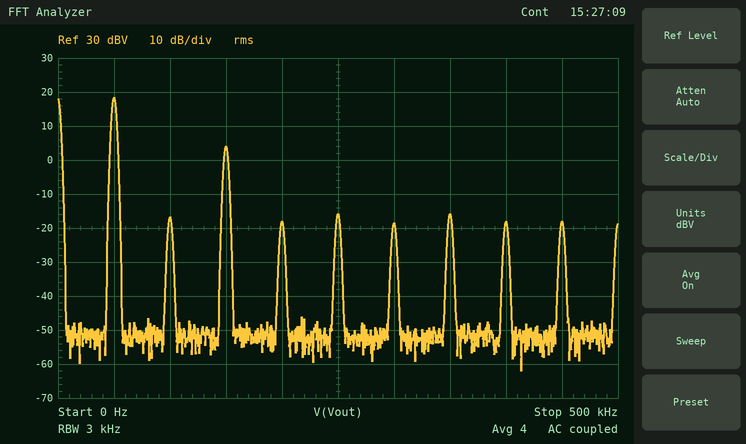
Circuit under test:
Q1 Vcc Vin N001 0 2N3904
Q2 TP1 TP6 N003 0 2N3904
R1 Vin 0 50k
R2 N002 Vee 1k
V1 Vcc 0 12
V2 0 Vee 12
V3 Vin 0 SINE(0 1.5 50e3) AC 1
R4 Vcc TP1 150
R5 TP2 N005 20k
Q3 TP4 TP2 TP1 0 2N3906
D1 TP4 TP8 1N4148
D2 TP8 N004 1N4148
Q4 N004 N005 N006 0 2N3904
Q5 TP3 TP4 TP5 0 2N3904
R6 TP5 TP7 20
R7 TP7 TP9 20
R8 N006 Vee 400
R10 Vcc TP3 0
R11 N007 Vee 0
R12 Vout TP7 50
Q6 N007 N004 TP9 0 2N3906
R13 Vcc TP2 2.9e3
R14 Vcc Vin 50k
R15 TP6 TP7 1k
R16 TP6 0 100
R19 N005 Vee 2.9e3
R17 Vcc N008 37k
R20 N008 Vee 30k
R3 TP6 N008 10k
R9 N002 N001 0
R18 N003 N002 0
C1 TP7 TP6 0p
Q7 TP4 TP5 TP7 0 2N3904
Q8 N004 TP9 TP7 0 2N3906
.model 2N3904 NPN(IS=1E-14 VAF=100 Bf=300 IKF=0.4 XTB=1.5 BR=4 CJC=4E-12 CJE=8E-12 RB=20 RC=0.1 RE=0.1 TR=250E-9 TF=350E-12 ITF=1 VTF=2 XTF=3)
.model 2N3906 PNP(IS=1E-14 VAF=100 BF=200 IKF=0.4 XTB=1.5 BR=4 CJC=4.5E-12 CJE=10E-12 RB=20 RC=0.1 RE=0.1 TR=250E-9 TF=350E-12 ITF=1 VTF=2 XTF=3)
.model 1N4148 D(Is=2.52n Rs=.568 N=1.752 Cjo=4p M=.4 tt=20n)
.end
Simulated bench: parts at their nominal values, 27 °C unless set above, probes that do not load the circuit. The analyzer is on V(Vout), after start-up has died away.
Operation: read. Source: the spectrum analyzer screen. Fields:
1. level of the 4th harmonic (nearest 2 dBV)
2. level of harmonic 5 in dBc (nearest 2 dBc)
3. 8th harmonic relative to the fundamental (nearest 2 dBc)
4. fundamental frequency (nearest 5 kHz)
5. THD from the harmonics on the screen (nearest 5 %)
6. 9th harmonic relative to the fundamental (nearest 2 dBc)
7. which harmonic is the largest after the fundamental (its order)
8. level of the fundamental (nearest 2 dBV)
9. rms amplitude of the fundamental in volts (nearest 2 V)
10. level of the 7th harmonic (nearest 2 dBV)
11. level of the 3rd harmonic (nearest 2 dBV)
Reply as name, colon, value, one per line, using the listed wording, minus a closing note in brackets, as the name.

level of the 4th harmonic: -18 dBV
level of harmonic 5 in dBc: -34 dBc
8th harmonic relative to the fundamental: -36 dBc
fundamental frequency: 50 kHz
THD from the harmonics on the screen: 20 %
9th harmonic relative to the fundamental: -36 dBc
which harmonic is the largest after the fundamental: 3
level of the fundamental: 18 dBV
rms amplitude of the fundamental in volts: 8 V
level of the 7th harmonic: -16 dBV
level of the 3rd harmonic: 4 dBV
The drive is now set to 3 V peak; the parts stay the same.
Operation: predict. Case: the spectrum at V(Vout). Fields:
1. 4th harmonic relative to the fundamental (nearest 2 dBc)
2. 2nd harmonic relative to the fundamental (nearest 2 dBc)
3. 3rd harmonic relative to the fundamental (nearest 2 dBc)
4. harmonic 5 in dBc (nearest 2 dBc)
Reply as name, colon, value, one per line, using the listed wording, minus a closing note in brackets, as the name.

4th harmonic relative to the fundamental: -26 dBc
2nd harmonic relative to the fundamental: -26 dBc
3rd harmonic relative to the fundamental: -10 dBc
harmonic 5 in dBc: -16 dBc
